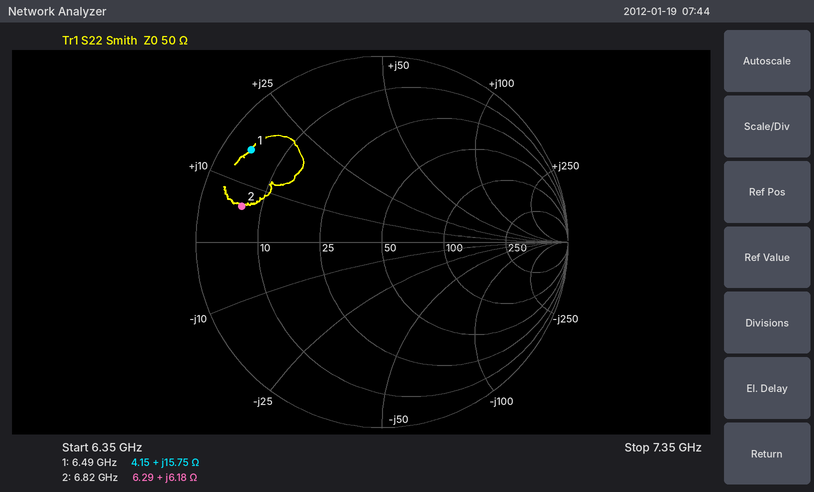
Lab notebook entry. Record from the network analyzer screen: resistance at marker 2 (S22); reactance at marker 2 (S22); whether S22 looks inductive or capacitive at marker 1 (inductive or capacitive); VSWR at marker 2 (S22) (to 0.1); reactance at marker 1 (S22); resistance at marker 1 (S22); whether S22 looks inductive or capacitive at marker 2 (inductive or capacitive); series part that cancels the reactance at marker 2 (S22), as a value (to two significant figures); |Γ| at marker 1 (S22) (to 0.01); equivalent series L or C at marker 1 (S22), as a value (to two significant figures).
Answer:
6.29 Ω
+6.18 Ω
inductive
8.1
+15.75 Ω
4.15 Ω
inductive
3.8 pF
0.86
390 pH
